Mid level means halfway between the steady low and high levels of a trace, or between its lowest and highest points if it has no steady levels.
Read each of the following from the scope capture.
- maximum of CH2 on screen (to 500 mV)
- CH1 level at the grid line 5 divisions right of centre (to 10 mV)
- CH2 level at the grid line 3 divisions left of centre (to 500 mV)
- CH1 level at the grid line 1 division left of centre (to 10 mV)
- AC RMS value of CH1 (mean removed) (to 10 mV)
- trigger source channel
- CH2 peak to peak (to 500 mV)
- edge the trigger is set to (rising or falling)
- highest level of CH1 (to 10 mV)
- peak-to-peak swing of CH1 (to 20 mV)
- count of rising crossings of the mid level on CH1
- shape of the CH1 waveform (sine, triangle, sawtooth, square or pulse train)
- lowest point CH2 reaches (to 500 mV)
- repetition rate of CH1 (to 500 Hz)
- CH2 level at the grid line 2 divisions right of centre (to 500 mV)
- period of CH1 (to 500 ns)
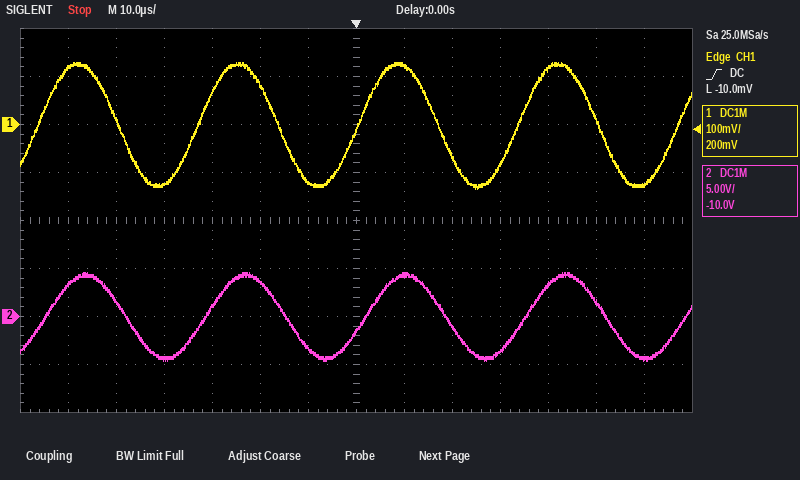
4.5 V
10 mV
1.0 V
-120 mV
90 mV
CH1
9.0 V
rising
130 mV
260 mV
5
sine
-4.5 V
30.0 kHz
-1.0 V
33.5 µs
